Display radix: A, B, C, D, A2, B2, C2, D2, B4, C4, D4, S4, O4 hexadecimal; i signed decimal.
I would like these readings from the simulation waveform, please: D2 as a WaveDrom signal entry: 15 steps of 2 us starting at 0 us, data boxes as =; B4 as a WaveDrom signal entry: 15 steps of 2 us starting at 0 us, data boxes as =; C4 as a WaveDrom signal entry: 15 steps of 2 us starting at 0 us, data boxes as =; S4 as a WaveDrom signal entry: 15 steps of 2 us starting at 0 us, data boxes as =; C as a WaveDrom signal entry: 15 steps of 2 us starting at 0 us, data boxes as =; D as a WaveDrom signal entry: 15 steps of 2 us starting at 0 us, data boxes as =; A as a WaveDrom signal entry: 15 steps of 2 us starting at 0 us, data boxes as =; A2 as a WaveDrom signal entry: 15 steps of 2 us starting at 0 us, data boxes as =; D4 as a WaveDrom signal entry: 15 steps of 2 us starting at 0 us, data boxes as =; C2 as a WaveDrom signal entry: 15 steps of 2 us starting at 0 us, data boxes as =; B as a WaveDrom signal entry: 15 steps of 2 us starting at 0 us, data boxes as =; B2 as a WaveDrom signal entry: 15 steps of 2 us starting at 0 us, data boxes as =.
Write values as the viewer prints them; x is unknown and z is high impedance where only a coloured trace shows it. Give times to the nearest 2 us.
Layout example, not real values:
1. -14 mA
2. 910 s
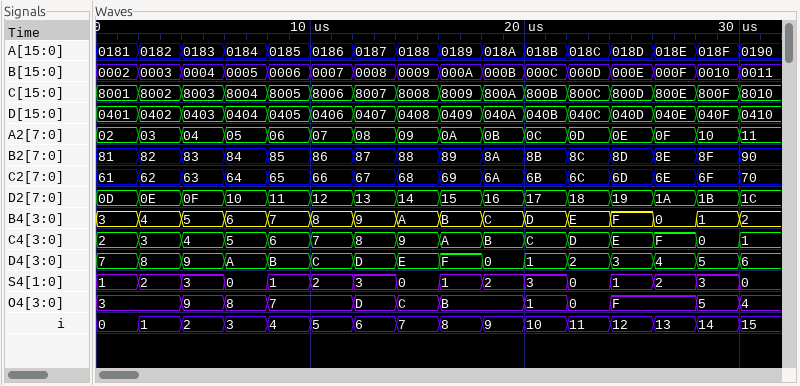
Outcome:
1. {name: 'D2', wave: '===============', data: '0D 0E 0F 10 11 12 13 14 15 16 17 18 19 1A 1B'}
2. {name: 'B4', wave: '===============', data: '3 4 5 6 7 8 9 A B C D E F 0 1'}
3. {name: 'C4', wave: '===============', data: '2 3 4 5 6 7 8 9 A B C D E F 0'}
4. {name: 'S4', wave: '===============', data: '1 2 3 0 1 2 3 0 1 2 3 0 1 2 3'}
5. {name: 'C', wave: '===============', data: '8001 8002 8003 8004 8005 8006 8007 8008 8009 800A 800B 800C 800D 800E 800F'}
6. {name: 'D', wave: '===============', data: '0401 0402 0403 0404 0405 0406 0407 0408 0409 040A 040B 040C 040D 040E 040F'}
7. {name: 'A', wave: '===============', data: '0181 0182 0183 0184 0185 0186 0187 0188 0189 018A 018B 018C 018D 018E 018F'}
8. {name: 'A2', wave: '===============', data: '02 03 04 05 06 07 08 09 0A 0B 0C 0D 0E 0F 10'}
9. {name: 'D4', wave: '===============', data: '7 8 9 A B C D E F 0 1 2 3 4 5'}
10. {name: 'C2', wave: '===============', data: '61 62 63 64 65 66 67 68 69 6A 6B 6C 6D 6E 6F'}
11. {name: 'B', wave: '===============', data: '0002 0003 0004 0005 0006 0007 0008 0009 000A 000B 000C 000D 000E 000F 0010'}
12. {name: 'B2', wave: '===============', data: '81 82 83 84 85 86 87 88 89 8A 8B 8C 8D 8E 8F'}
